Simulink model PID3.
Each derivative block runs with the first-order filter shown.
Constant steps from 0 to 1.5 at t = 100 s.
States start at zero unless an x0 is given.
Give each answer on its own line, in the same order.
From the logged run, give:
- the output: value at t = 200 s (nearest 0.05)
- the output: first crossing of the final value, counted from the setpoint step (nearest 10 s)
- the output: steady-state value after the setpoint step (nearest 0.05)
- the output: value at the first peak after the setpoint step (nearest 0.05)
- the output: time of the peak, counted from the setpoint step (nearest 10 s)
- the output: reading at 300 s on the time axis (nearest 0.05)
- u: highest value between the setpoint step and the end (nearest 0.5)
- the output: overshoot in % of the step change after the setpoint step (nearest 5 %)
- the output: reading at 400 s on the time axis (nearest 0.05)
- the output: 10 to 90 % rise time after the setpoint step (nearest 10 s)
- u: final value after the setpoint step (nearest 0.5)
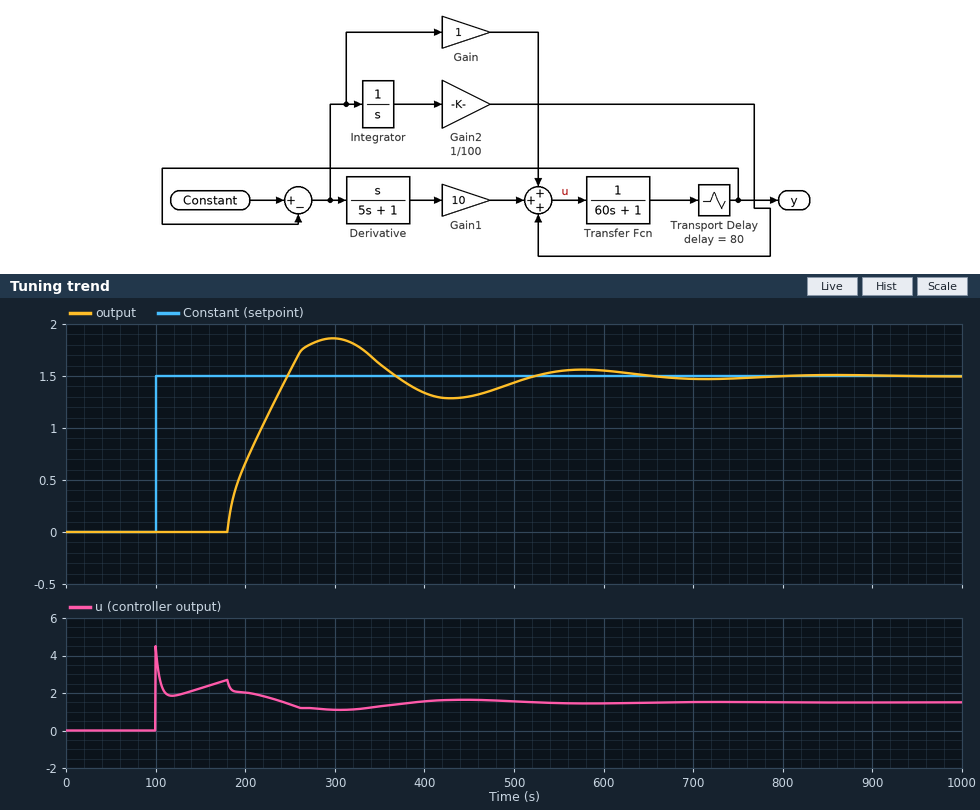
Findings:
0.65
150 s
1.50
1.85
200 s
1.85
4.5
25 %
1.35
60 s
1.5
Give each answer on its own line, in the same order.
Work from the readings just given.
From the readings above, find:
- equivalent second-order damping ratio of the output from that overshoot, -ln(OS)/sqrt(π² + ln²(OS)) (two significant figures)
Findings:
0.40
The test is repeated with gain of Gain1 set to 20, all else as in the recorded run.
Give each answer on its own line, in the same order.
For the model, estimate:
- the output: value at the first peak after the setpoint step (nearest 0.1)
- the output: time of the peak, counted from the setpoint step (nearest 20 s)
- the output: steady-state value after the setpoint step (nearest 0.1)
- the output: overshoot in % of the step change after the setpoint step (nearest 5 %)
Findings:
1.8
160 s
1.5
20 %
